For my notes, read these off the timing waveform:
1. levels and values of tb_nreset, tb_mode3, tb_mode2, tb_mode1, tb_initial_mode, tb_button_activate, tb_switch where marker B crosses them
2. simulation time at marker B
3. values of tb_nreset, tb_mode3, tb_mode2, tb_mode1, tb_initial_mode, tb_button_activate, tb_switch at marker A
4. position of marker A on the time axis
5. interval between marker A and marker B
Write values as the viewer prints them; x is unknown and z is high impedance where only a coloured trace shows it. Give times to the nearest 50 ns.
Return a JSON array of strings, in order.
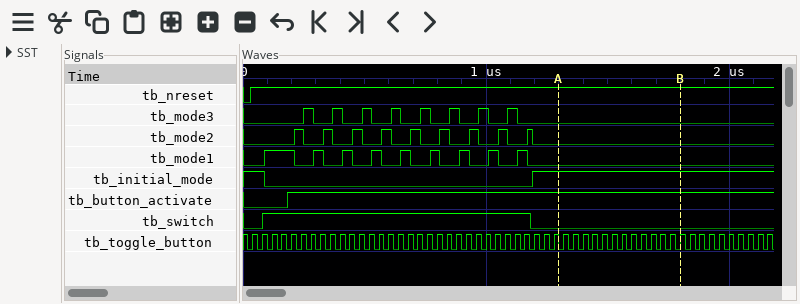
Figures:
["tb_nreset=1, tb_mode3=0, tb_mode2=0, tb_mode1=0, tb_initial_mode=1, tb_button_activate=1, tb_switch=0", "1800 ns", "tb_nreset=1, tb_mode3=0, tb_mode2=0, tb_mode1=0, tb_initial_mode=1, tb_button_activate=1, tb_switch=0", "1300 ns", "500 ns"]
